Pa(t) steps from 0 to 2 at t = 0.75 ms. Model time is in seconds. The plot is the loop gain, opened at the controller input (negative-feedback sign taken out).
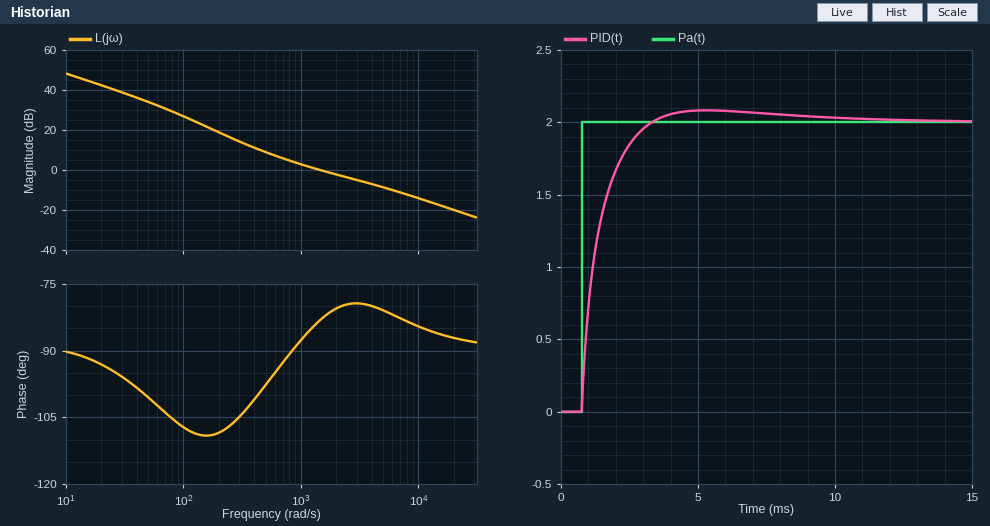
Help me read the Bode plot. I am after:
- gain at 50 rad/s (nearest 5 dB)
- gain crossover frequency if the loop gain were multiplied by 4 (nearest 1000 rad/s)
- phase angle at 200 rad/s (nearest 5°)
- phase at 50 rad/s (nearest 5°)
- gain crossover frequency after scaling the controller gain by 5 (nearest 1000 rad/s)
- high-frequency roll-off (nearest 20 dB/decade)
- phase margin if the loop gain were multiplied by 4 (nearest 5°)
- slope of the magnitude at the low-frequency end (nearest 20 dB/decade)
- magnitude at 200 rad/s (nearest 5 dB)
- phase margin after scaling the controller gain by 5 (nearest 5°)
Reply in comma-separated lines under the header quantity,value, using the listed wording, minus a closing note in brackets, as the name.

quantity,value
gain at 50 rad/s,35 dB
gain crossover frequency if the loop gain were multiplied by 4,8000 rad/s
phase angle at 200 rad/s,-110°
phase at 50 rad/s,-100°
gain crossover frequency after scaling the controller gain by 5,10000 rad/s
high-frequency roll-off,-20 dB/decade
phase margin if the loop gain were multiplied by 4,95°
slope of the magnitude at the low-frequency end,-20 dB/decade
magnitude at 200 rad/s,20 dB
phase margin after scaling the controller gain by 5,95°
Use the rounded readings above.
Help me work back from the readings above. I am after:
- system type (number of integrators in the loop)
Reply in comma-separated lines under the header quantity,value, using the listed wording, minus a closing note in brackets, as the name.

quantity,value
system type,1
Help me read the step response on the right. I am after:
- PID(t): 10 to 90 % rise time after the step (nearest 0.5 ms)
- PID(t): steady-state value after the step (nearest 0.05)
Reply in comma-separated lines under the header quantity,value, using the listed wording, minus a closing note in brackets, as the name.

quantity,value
PID(t): 10 to 90 % rise time after the step,1.5 ms
PID(t): steady-state value after the step,2.00
